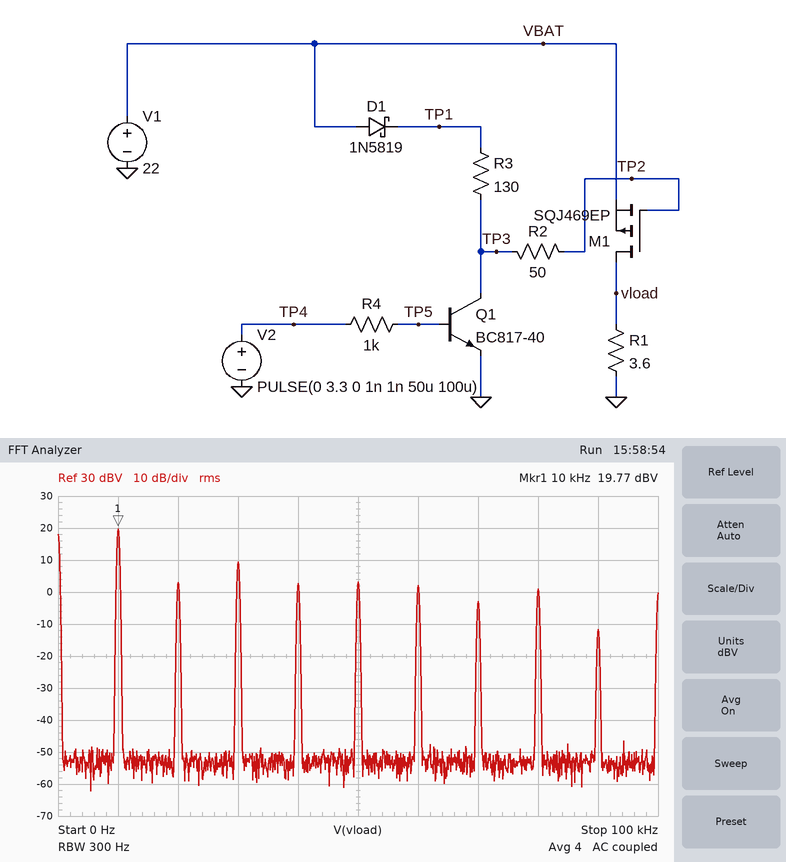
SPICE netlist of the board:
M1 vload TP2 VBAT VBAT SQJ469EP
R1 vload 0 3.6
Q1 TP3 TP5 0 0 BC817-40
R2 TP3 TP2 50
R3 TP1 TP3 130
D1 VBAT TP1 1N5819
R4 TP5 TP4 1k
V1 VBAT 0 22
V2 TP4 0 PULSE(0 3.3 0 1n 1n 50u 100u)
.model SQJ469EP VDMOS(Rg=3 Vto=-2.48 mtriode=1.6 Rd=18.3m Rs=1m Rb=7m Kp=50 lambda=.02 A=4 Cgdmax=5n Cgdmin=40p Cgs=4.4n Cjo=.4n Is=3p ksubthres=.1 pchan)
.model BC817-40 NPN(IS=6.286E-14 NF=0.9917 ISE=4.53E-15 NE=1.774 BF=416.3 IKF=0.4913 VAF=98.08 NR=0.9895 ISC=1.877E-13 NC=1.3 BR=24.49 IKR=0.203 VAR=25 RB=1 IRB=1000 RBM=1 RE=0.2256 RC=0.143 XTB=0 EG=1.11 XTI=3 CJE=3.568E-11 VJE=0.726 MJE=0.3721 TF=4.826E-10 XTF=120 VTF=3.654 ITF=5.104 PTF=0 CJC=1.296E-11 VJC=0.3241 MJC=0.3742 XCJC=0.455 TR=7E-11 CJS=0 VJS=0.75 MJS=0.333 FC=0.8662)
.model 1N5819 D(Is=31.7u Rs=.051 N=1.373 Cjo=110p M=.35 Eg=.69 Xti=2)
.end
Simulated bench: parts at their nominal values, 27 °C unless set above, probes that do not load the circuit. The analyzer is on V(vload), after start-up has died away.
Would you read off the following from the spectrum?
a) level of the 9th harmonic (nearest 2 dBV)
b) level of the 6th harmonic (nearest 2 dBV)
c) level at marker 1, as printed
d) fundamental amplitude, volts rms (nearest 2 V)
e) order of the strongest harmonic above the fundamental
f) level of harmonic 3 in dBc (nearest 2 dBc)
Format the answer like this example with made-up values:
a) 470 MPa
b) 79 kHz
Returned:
a) -12 dBV
b) 2 dBV
c) 19.77 dBV
d) 10 V
e) 3
f) -10 dBc
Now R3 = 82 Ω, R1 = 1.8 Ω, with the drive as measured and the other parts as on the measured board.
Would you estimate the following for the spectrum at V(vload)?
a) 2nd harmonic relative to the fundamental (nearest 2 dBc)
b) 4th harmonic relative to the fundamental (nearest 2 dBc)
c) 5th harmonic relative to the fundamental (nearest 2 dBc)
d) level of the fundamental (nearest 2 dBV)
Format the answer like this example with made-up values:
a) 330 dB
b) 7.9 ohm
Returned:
a) -20 dBc
b) -20 dBc
c) -16 dBc
d) 20 dBV
